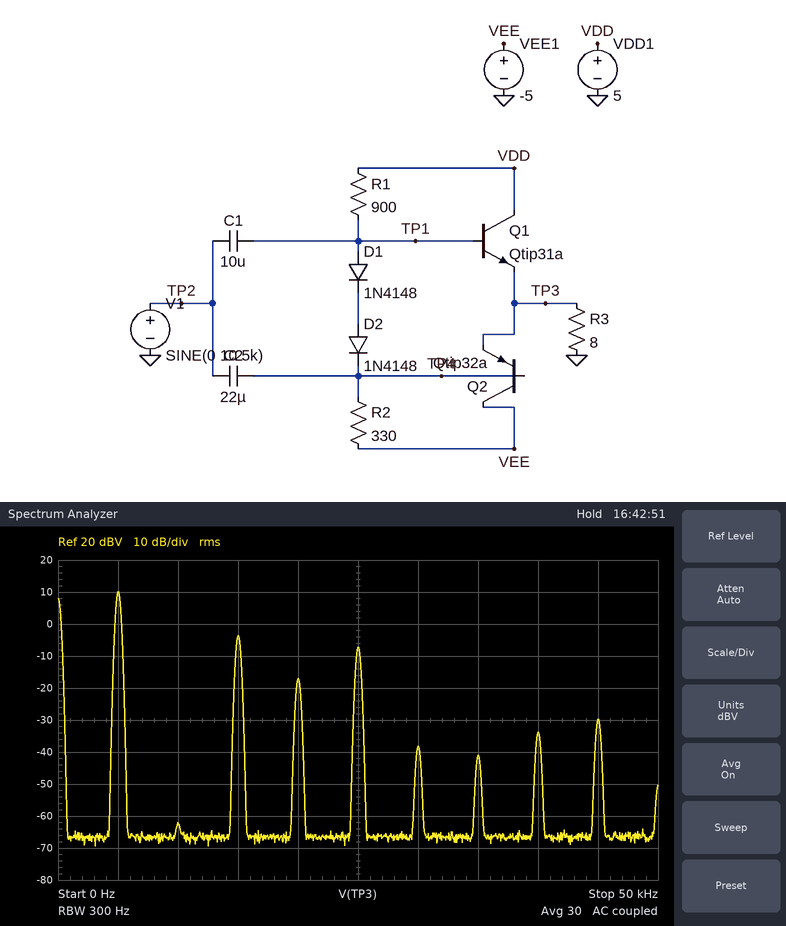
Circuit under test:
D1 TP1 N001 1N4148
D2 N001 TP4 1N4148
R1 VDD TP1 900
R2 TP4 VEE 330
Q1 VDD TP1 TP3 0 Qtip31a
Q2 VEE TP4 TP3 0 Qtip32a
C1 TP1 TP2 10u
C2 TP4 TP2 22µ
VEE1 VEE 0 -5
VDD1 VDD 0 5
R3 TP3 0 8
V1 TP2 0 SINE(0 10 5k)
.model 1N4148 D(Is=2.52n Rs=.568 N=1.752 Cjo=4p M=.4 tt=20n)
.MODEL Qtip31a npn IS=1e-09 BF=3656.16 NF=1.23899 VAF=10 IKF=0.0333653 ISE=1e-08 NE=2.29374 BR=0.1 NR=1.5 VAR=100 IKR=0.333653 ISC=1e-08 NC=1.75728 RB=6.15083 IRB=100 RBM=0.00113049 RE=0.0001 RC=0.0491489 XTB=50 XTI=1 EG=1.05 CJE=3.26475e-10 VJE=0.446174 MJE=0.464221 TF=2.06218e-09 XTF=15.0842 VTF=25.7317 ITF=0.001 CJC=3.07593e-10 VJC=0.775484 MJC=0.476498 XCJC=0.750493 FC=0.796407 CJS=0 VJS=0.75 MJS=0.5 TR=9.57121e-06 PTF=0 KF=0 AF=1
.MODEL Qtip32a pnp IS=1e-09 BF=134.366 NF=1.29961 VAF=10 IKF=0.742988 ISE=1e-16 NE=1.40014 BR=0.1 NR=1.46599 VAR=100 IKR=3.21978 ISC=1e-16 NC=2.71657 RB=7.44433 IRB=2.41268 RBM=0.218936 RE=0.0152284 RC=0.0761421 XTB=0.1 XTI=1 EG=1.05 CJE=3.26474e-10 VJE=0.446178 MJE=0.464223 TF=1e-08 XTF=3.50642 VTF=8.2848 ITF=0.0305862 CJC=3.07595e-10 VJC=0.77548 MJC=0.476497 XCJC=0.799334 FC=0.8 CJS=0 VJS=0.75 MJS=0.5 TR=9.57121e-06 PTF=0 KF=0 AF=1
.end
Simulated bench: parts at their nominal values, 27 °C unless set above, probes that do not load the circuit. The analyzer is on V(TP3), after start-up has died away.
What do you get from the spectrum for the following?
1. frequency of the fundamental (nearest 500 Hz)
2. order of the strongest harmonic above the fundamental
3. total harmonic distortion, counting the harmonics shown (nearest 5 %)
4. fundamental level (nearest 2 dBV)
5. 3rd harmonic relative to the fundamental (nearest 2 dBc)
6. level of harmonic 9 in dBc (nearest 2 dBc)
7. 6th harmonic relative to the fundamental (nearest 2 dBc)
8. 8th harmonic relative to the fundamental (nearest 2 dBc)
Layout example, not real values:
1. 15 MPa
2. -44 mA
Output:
1. 5.0 kHz
2. 3
3. 25 %
4. 10 dBV
5. -14 dBc
6. -40 dBc
7. -48 dBc
8. -44 dBc
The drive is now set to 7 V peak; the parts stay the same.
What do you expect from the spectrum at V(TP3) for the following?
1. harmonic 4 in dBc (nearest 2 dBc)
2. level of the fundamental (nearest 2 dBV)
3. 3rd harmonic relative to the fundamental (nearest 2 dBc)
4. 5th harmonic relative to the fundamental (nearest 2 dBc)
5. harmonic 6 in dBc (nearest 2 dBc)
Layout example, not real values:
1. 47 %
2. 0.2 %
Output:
1. -32 dBc
2. 10 dBV
3. -24 dBc
4. -22 dBc
5. -46 dBc
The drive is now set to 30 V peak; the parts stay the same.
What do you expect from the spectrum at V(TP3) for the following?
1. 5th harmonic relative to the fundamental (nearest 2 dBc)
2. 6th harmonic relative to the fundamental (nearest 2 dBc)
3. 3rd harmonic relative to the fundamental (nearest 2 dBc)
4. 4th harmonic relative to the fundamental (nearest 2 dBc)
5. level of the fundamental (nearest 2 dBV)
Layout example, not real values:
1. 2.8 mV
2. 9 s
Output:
1. -32 dBc
2. -24 dBc
3. -6 dBc
4. -24 dBc
5. 8 dBV
